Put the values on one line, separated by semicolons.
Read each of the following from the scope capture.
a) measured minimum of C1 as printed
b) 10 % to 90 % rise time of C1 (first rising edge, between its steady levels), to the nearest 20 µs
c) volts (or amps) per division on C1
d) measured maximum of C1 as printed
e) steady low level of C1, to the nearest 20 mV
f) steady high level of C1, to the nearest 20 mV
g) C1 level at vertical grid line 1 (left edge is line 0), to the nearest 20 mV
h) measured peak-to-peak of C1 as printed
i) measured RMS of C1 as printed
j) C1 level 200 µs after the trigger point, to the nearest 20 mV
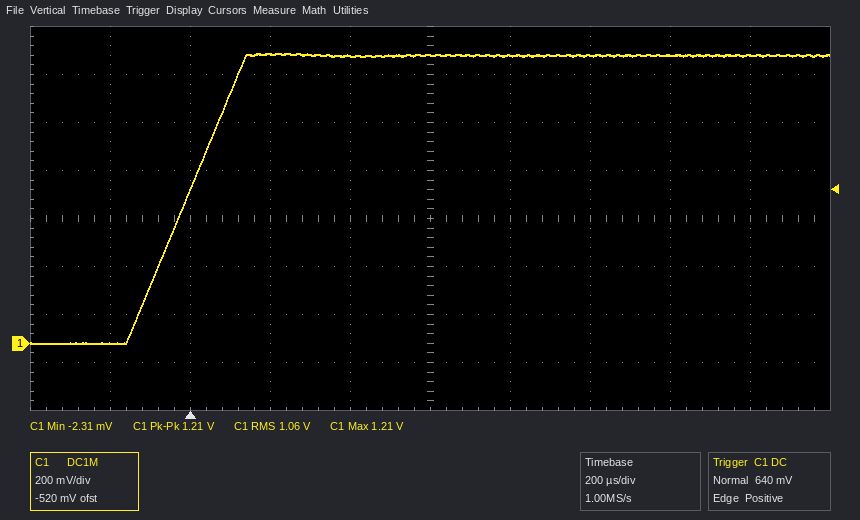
-2.31 mV; 240 µs; 200 mV; 1.21 V; 0 mV; 1.20 V; 0 mV; 1.21 V; 1.06 V; 1.20 V
